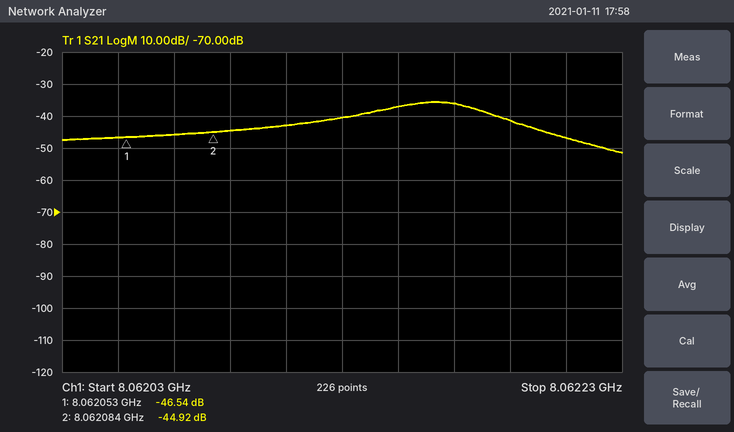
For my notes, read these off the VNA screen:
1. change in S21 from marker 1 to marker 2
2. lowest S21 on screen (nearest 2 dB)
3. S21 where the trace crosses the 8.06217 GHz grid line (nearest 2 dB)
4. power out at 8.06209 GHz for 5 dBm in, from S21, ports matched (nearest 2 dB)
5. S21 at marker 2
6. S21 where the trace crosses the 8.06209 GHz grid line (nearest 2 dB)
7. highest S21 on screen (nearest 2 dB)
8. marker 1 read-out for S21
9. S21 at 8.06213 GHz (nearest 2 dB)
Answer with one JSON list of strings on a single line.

["1.62 dB", "-52 dB", "-36 dB", "-40 dBm", "-44.92 dB", "-44 dB", "-36 dB", "-46.54 dB", "-40 dB"]
